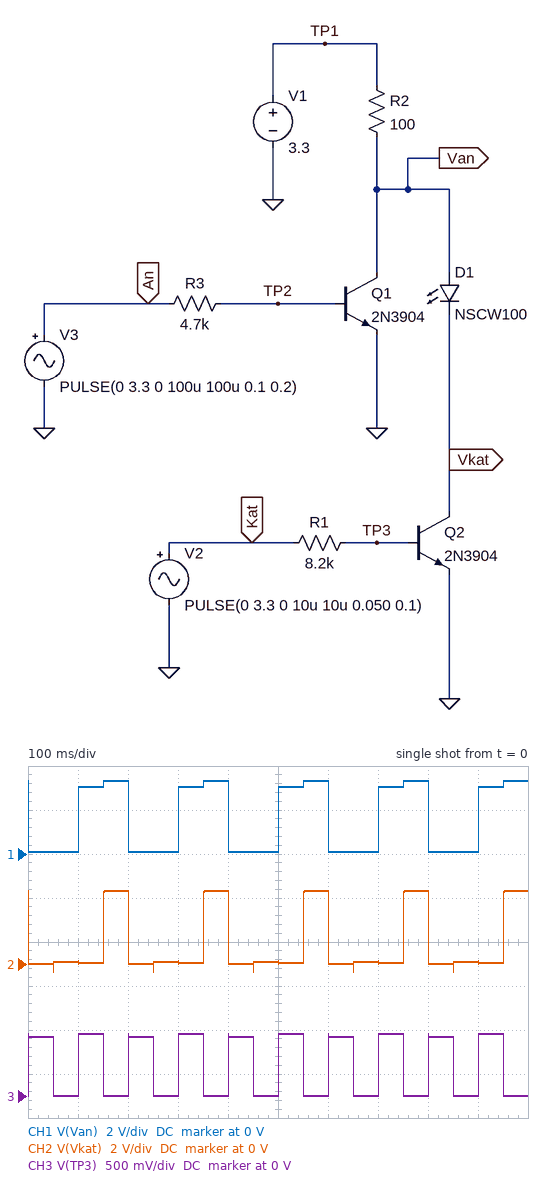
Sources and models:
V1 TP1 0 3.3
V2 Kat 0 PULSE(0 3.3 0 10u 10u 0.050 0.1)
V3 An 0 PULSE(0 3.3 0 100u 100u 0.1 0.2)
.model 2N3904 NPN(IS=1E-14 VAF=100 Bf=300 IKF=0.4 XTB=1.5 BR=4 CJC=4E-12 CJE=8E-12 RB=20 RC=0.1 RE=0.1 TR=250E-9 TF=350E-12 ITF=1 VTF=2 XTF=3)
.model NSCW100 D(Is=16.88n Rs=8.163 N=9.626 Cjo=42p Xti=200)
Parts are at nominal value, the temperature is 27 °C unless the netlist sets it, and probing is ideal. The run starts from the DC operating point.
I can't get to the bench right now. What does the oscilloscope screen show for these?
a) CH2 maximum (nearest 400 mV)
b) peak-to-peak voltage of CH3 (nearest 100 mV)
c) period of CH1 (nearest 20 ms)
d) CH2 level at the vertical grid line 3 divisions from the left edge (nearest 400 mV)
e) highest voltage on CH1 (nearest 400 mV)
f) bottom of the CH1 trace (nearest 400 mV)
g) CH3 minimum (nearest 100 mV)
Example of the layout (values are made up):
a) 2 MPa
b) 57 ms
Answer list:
a) 3.2 V
b) 700 mV
c) 200 ms
d) 0 V
e) 3.2 V
f) 0 V
g) 0 V
